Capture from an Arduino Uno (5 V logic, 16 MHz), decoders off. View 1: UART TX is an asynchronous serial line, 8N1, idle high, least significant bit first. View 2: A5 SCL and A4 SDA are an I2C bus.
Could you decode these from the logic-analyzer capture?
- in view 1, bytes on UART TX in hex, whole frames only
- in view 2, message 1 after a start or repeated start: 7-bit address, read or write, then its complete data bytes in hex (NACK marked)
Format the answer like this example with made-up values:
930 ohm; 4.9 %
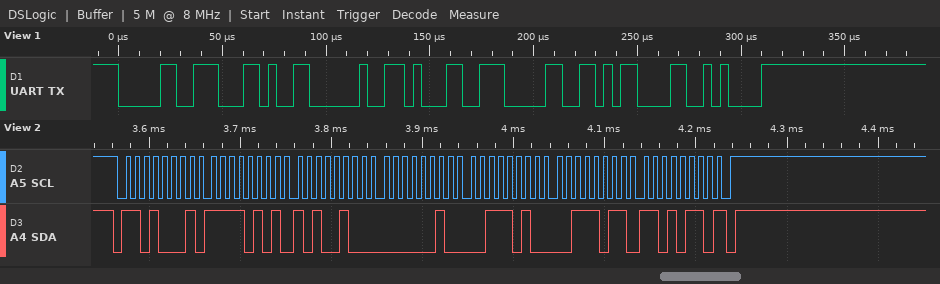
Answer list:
30 2C 20 31 30 0D 0A; 0x68 read: F5 A4 02 3A 3B D6 NACK
